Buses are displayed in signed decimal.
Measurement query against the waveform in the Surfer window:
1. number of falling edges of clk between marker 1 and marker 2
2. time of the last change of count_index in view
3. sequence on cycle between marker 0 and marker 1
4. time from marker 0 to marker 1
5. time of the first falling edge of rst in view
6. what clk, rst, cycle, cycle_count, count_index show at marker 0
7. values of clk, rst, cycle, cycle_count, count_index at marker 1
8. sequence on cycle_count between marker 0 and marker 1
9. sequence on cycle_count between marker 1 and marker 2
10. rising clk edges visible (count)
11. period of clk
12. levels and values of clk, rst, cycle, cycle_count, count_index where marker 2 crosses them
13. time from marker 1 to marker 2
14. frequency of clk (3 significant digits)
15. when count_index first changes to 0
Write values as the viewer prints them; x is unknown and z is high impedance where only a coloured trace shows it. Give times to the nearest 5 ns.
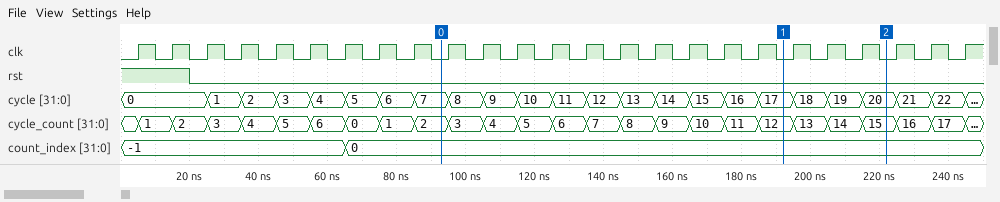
3
65 ns
7, 8, 9, 10, 11, 12, 13, 14, 15, 16, 17
100 ns
20 ns
clk=0, rst=0, cycle=7, cycle_count=2, count_index=0
clk=0, rst=0, cycle=17, cycle_count=12, count_index=0
2, 3, 4, 5, 6, 7, 8, 9, 10, 11, 12
12, 13, 14, 15
25
10 ns
clk=0, rst=0, cycle=20, cycle_count=15, count_index=0
30 ns
100 MHz
65 ns
